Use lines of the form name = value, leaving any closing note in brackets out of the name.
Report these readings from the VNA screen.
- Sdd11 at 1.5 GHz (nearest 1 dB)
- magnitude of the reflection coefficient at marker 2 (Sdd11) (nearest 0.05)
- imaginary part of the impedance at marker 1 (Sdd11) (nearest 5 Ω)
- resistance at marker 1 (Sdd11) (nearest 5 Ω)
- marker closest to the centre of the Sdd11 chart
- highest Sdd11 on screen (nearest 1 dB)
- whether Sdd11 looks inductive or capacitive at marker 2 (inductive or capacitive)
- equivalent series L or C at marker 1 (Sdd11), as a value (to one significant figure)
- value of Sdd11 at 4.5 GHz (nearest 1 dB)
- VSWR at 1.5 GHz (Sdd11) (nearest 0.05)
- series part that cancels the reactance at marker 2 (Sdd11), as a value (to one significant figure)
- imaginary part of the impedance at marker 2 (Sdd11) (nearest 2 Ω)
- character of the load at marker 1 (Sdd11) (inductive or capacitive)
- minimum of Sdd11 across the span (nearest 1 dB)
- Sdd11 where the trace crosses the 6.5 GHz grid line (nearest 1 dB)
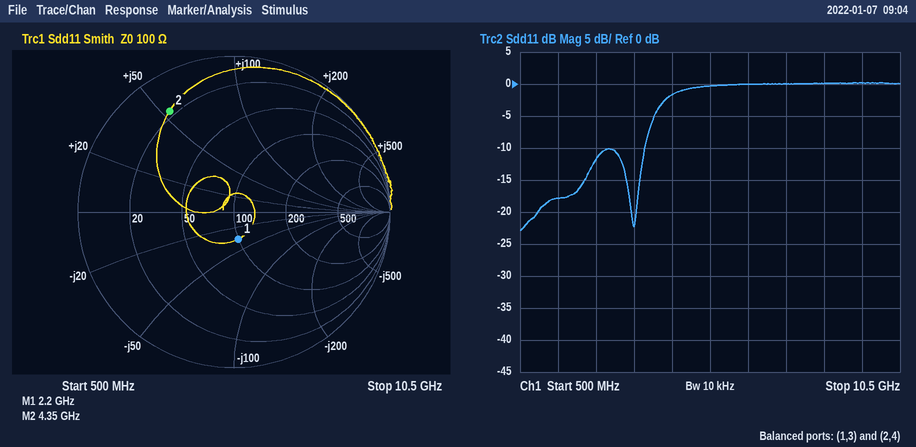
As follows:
Sdd11 at 1.5 GHz = -18 dB
magnitude of the reflection coefficient at marker 2 (Sdd11) = 0.75
imaginary part of the impedance at marker 1 (Sdd11) = -35 Ω
resistance at marker 1 (Sdd11) = 100 Ω
marker closest to the centre of the Sdd11 chart = marker 1
highest Sdd11 on screen = 0 dB
whether Sdd11 looks inductive or capacitive at marker 2 = inductive
equivalent series L or C at marker 1 (Sdd11), as a value = 2 pF
value of Sdd11 at 4.5 GHz = -2 dB
VSWR at 1.5 GHz (Sdd11) = 1.30
series part that cancels the reactance at marker 2 (Sdd11), as a value = 700 fF
imaginary part of the impedance at marker 2 (Sdd11) = +54 Ω
character of the load at marker 1 (Sdd11) = capacitive
minimum of Sdd11 across the span = -23 dB
Sdd11 where the trace crosses the 6.5 GHz grid line = 0 dB
